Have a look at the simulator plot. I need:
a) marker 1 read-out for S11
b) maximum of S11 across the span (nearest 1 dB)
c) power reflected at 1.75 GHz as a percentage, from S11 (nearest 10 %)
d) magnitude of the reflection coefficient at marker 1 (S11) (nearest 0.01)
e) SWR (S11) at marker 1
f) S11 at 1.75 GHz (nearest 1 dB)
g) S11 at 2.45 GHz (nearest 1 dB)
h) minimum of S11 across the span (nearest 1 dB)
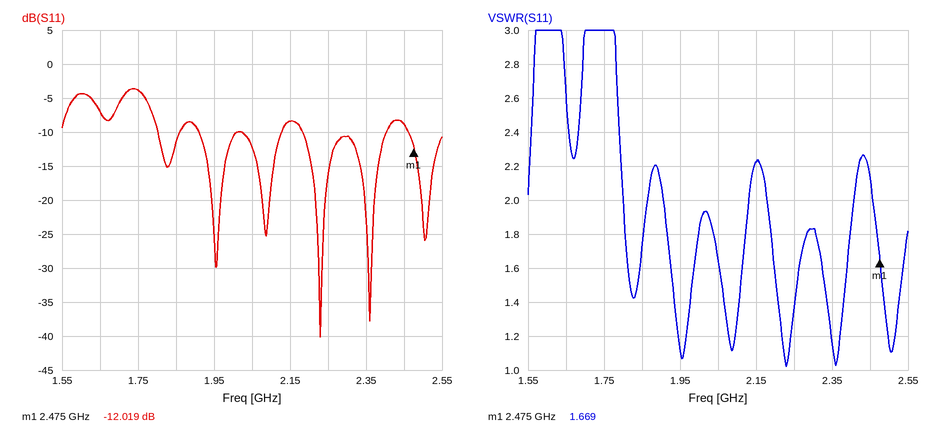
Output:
-12.019 dB
-4 dB
40 %
0.25
1.669
-4 dB
-9 dB
-40 dB
